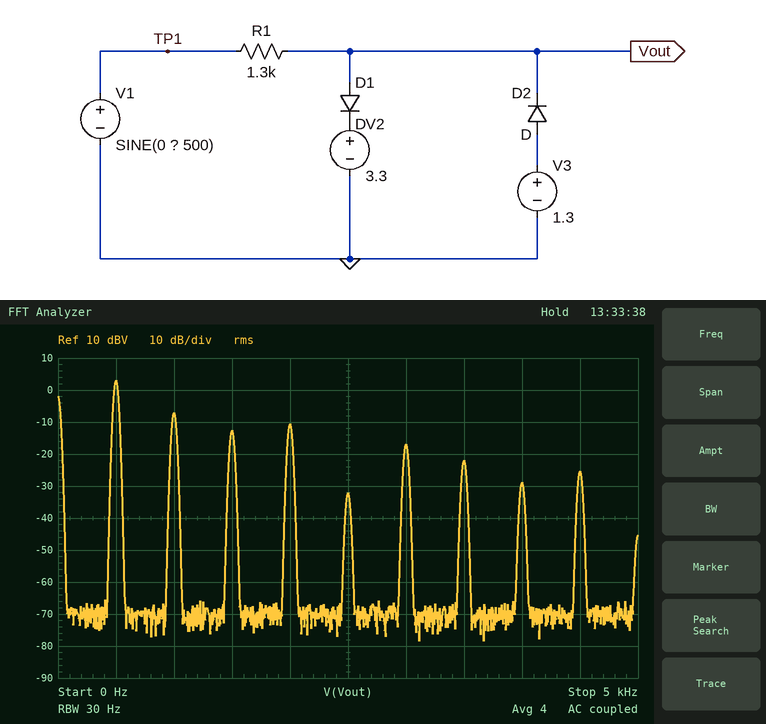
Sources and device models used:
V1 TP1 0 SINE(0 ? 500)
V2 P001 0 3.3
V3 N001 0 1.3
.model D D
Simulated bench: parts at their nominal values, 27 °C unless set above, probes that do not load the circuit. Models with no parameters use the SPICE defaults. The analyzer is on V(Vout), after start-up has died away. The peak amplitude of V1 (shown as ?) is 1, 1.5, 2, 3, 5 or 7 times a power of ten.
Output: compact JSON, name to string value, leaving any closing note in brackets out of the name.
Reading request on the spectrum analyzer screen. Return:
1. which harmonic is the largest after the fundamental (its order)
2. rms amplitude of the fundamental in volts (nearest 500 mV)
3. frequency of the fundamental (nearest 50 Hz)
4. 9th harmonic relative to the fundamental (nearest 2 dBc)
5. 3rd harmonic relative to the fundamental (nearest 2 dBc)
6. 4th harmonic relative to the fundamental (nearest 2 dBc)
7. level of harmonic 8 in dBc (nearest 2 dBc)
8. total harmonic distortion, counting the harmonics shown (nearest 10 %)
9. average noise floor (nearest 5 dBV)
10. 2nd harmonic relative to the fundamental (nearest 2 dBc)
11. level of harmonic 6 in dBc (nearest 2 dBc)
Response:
{"which harmonic is the largest after the fundamental": "2", "rms amplitude of the fundamental in volts": "1.5 V", "frequency of the fundamental": "500 Hz", "9th harmonic relative to the fundamental": "-28 dBc", "3rd harmonic relative to the fundamental": "-16 dBc", "4th harmonic relative to the fundamental": "-14 dBc", "level of harmonic 8 in dBc": "-32 dBc", "total harmonic distortion, counting the harmonics shown": "40 %", "average noise floor": "-70 dBV", "2nd harmonic relative to the fundamental": "-10 dBc", "level of harmonic 6 in dBc": "-20 dBc"}
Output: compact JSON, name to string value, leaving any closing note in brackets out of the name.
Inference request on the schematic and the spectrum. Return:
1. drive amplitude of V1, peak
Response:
{"drive amplitude of V1, peak": "7 V"}
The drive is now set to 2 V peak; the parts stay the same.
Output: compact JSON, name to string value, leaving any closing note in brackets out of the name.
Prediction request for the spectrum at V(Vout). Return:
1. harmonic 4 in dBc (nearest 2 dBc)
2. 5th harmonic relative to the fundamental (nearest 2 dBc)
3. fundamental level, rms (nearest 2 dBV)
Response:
{"harmonic 4 in dBc": "-30 dBc", "5th harmonic relative to the fundamental": "-22 dBc", "fundamental level, rms": "-8 dBV"}
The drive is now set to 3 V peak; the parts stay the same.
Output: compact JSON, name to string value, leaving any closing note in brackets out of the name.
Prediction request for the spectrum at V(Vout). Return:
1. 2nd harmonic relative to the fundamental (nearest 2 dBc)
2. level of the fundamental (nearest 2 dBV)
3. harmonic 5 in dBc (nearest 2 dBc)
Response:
{"2nd harmonic relative to the fundamental": "-6 dBc", "level of the fundamental": "-2 dBV", "harmonic 5 in dBc": "-24 dBc"}
